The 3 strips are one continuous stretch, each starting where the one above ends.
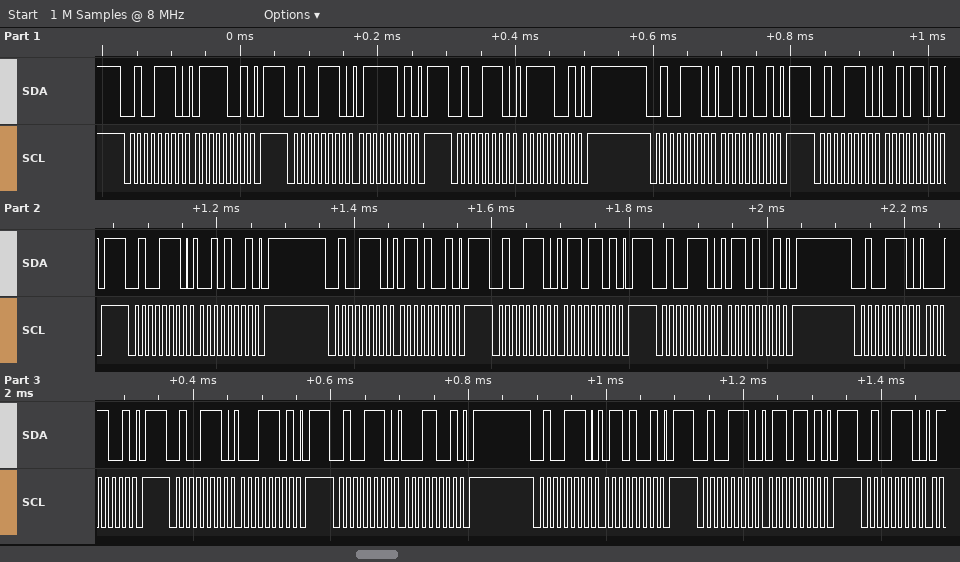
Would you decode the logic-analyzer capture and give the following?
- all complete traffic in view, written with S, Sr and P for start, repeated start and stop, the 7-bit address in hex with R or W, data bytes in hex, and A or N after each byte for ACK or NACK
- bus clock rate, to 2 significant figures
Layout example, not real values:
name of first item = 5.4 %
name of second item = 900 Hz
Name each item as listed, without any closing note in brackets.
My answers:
all complete traffic in view, written with S, Sr and P for start, repeated start and stop, the 7-bit address in hex with R or W, data bytes in hex, and A or N after each byte for ACK or NACK = S 27W A 79 A P S 27W A 7D A P S 27W A 79 A P S 27W A 29 A P S 27W A 2D A P S 27W A 29 A P S 27W A 69 A P S 27W A 6D A P S 27W A 69 A P S 27W A 19 A P S 27W A 1D A P S 27W A 19 A P S 27W A 69 A P S 27W A 6D A P S 27W A
bus clock rate, to 2 significant figures = 100 kHz
